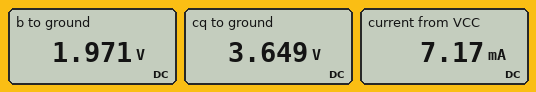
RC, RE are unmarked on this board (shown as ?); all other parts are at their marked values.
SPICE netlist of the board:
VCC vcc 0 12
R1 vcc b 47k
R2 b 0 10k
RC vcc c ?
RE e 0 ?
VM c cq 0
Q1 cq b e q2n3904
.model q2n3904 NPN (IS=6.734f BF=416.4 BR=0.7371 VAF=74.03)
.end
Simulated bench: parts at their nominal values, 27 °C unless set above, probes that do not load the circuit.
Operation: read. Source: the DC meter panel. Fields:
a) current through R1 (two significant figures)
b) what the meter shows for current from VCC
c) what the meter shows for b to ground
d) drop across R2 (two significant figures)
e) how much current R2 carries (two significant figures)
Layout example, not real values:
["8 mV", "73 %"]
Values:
["210 µA", "7.17 mA", "1.971 V", "2.0 V", "200 µA"]
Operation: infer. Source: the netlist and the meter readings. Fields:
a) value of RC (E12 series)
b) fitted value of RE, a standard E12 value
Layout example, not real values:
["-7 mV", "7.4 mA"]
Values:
["1.2 kΩ", "180 Ω"]
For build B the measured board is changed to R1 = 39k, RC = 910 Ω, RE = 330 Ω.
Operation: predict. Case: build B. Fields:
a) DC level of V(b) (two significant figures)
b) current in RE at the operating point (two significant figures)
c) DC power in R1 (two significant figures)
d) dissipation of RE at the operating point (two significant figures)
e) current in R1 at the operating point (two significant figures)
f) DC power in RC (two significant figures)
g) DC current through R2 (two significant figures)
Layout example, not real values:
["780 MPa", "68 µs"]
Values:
["2.4 V", "5.0 mA", "2.4 mW", "8.3 mW", "250 µA", "23 mW", "240 µA"]
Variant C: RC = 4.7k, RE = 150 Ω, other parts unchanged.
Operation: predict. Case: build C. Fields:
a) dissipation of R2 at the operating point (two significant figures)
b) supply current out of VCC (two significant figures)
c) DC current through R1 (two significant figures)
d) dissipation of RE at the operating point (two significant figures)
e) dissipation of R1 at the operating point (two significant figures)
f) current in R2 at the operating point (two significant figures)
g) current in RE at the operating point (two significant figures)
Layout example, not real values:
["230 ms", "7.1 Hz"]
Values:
["120 µW", "2.7 mA", "230 µA", "1.0 mW", "2.5 mW", "110 µA", "2.6 mA"]
